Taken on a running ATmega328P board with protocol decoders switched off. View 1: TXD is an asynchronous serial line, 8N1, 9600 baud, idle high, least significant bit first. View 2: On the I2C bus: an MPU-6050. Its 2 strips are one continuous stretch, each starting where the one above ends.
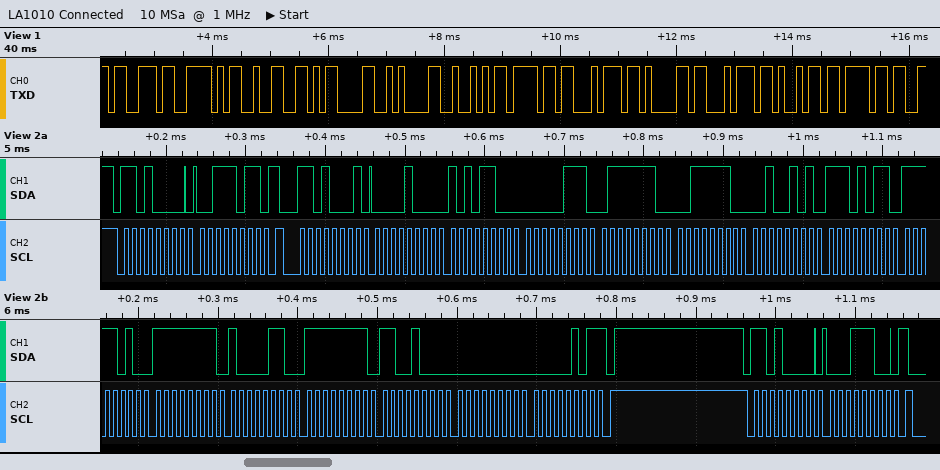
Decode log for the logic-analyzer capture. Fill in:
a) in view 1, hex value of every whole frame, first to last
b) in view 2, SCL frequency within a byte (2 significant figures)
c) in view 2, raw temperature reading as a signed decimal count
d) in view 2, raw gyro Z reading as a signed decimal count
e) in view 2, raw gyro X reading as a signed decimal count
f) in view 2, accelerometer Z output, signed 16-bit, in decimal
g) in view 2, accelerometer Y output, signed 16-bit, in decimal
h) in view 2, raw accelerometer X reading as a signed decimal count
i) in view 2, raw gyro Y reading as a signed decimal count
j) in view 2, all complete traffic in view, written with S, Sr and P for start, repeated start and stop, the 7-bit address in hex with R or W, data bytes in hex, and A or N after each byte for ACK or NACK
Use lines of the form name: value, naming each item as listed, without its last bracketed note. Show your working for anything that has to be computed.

in view 1, hex value of every whole frame, first to last: 73 5E 32 0D 0A 52 6F 74 61 74 69 6F
in view 2, SCL frequency within a byte: 100 kHz
in view 2, raw temperature reading as a signed decimal count: 0xEBFA = -5126
in view 2, raw gyro Z reading as a signed decimal count: 0x0005 = 5
in view 2, raw gyro X reading as a signed decimal count: 0xFF86 = -122
in view 2, accelerometer Z output, signed 16-bit, in decimal: 0x3E25 = 15909
in view 2, accelerometer Y output, signed 16-bit, in decimal: 0x077E = 1918
in view 2, raw accelerometer X reading as a signed decimal count: 0x08AC = 2220
in view 2, raw gyro Y reading as a signed decimal count: 0xFFC8 = -56
in view 2, all complete traffic in view, written with S, Sr and P for start, repeated start and stop, the 7-bit address in hex with R or W, data bytes in hex, and A or N after each byte for ACK or NACK: S 68W A 3B A Sr 68R A 08 A AC A 07 A 7E A 3E A 25 A EB A FA A FF A 86 A FF A C8 A 00 A 05 N P S 68W A 1C A
